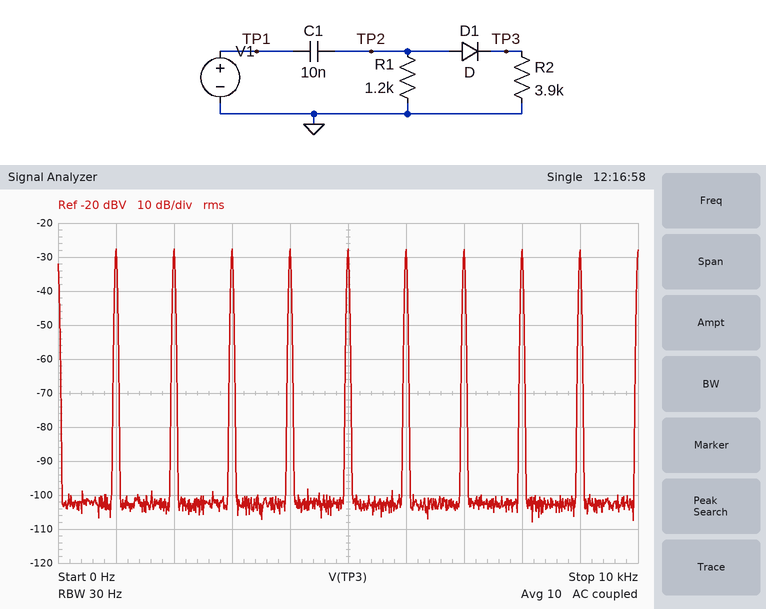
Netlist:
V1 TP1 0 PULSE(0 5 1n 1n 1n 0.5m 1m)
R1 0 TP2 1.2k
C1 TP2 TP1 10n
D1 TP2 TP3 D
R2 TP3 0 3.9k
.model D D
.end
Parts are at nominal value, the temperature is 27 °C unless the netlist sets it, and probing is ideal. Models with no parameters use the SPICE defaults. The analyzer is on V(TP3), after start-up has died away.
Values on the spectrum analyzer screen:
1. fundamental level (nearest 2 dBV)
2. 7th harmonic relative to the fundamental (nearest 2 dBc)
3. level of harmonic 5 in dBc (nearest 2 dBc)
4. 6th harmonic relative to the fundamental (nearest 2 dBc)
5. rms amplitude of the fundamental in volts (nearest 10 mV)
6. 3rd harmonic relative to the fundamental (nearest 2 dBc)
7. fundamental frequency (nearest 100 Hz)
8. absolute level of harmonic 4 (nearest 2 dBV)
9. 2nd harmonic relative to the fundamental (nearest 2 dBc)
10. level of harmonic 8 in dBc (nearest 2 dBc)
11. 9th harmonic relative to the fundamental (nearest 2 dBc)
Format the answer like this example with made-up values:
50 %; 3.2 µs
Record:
-28 dBV; 0 dBc; 0 dBc; 0 dBc; 40 mV; 0 dBc; 1.0 kHz; -28 dBV; 0 dBc; 0 dBc; 0 dBc
